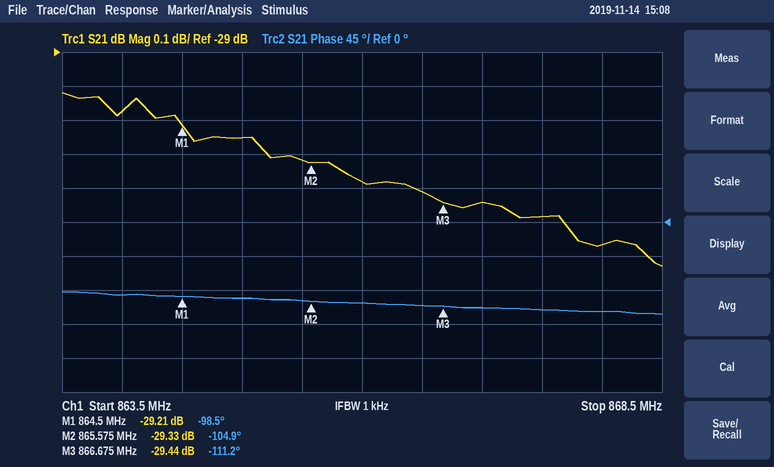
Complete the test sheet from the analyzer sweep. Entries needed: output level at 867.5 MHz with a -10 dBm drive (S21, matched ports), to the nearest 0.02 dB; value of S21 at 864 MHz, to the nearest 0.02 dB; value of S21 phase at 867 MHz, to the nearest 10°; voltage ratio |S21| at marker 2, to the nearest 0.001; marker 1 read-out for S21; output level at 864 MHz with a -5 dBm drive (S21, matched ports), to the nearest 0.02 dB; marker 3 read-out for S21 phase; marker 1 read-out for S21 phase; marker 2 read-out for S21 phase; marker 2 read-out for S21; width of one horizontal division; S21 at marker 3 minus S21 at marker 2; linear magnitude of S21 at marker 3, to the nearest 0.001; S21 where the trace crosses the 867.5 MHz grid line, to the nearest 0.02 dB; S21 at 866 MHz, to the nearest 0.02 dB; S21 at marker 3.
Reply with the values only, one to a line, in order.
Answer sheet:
-39.48 dBm
-29.18 dB
-110°
0.034
-29.21 dB
-34.18 dBm
-111.2°
-98.5°
-104.9°
-29.33 dB
500 kHz
-0.11 dB
0.034
-29.48 dB
-29.38 dB
-29.44 dB
